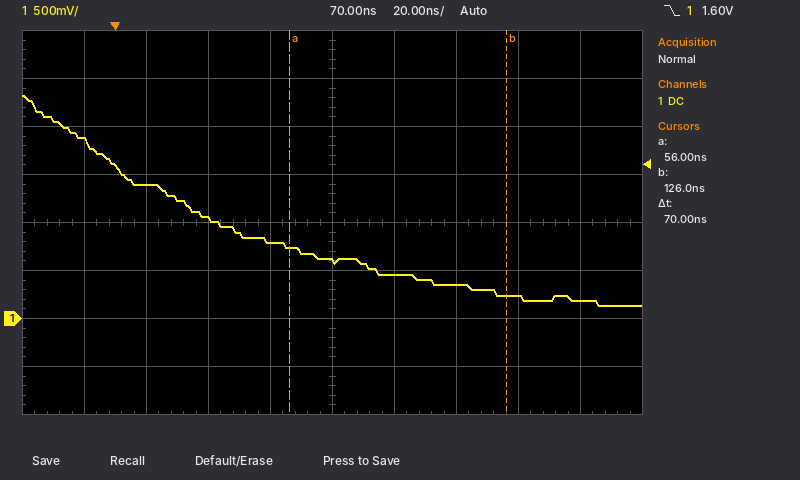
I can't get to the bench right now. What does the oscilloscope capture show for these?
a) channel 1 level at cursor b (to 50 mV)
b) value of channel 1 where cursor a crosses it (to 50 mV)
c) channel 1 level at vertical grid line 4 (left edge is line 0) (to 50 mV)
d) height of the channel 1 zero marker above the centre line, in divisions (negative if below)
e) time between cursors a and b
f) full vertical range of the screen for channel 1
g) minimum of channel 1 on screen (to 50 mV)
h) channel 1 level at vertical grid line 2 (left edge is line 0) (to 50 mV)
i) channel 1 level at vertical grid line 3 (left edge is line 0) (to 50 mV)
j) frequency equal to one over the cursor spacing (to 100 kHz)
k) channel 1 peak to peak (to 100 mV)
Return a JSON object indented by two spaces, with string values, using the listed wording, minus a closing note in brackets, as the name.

{
  "channel 1 level at cursor b": "250 mV",
  "value of channel 1 where cursor a crosses it": "750 mV",
  "channel 1 level at vertical grid line 4 (left edge is line 0)": "800 mV",
  "height of the channel 1 zero marker above the centre line, in divisions": "-2.0 div",
  "time between cursors a and b": "70 ns",
  "full vertical range of the screen for channel 1": "4 V",
  "minimum of channel 1 on screen": "150 mV",
  "channel 1 level at vertical grid line 2 (left edge is line 0)": "1.40 V",
  "channel 1 level at vertical grid line 3 (left edge is line 0)": "1.05 V",
  "frequency equal to one over the cursor spacing": "14.3 MHz",
  "channel 1 peak to peak": "2.20 V"
}
